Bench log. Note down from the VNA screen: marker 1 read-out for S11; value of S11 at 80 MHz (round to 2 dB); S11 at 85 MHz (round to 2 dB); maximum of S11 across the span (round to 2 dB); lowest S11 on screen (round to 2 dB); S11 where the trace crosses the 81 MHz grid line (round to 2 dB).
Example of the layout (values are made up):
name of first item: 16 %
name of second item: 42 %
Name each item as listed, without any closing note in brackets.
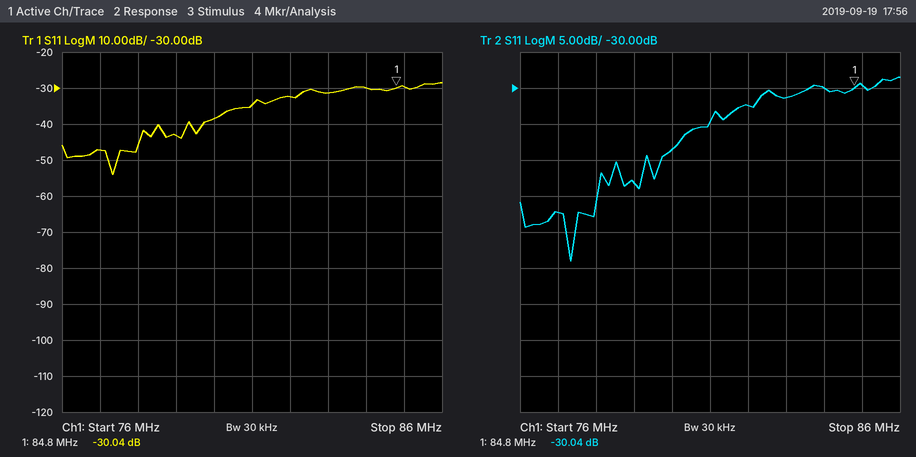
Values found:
marker 1 read-out for S11: -30.04 dB
value of S11 at 80 MHz: -38 dB
S11 at 85 MHz: -30 dB
maximum of S11 across the span: -28 dB
lowest S11 on screen: -54 dB
S11 where the trace crosses the 81 MHz grid line: -34 dB
